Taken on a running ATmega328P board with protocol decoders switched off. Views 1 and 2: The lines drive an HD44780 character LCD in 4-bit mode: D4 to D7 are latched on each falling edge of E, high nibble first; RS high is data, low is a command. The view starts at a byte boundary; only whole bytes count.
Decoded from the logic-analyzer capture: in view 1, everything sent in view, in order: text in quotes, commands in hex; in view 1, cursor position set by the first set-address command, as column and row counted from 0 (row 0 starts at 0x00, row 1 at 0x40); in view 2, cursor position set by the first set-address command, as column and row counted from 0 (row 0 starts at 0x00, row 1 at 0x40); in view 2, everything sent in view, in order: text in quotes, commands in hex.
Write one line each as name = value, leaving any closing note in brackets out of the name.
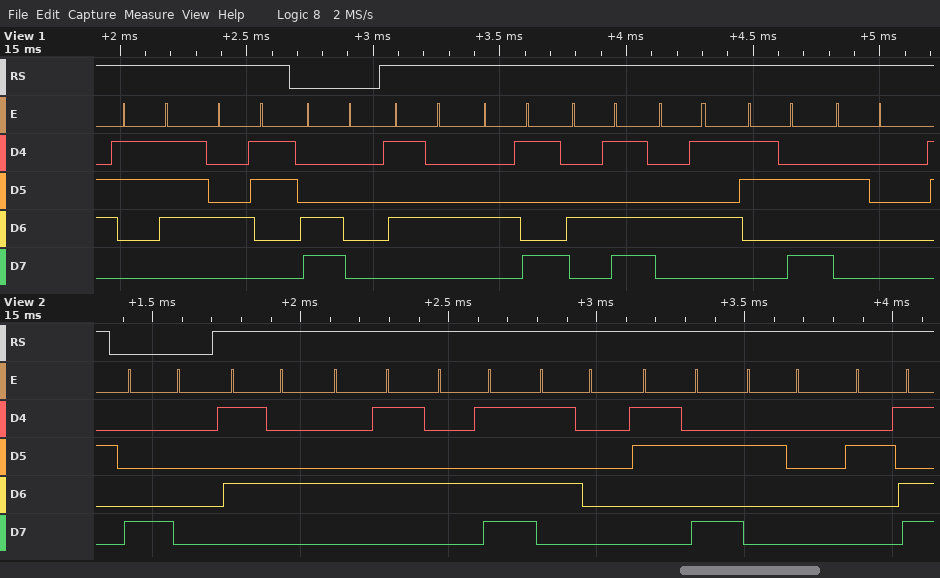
in view 1, everything sent in view, in order: text in quotes, commands in hex = "7C" 0xC0 "TIME: "
in view 1, cursor position set by the first set-address command, as column and row counted from 0 = column 0, row 1
in view 2, cursor position set by the first set-address command, as column and row counted from 0 = column 0, row 0
in view 2, everything sent in view, in order: text in quotes, commands in hex = 0x80 "TEMP: -"
